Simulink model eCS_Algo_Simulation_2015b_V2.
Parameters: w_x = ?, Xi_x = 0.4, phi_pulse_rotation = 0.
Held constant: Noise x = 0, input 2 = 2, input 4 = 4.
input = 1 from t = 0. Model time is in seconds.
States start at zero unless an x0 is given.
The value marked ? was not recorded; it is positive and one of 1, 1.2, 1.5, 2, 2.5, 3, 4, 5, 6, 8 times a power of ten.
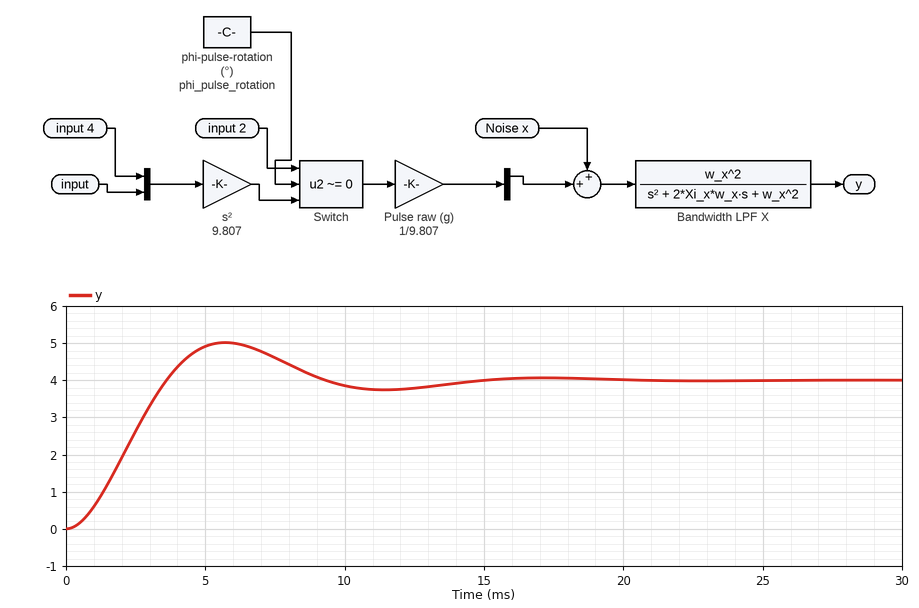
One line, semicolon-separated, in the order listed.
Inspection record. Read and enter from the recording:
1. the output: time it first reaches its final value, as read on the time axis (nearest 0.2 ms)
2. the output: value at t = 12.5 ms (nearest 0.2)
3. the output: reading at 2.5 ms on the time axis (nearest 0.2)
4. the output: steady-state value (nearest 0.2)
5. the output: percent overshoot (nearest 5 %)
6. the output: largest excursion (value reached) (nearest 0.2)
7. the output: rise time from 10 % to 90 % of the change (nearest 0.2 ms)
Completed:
3.6 ms; 3.8; 2.6; 4.0; 25 %; 5.0; 2.4 ms
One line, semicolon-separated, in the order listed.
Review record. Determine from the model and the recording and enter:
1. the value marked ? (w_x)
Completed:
600
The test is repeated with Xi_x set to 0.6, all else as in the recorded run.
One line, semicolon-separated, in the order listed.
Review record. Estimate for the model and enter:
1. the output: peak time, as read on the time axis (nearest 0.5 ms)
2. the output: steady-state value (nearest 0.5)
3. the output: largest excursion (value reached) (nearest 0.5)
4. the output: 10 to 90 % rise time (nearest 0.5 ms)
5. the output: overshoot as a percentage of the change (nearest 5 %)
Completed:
6.5 ms; 4.0; 4.5; 3.0 ms; 10 %
